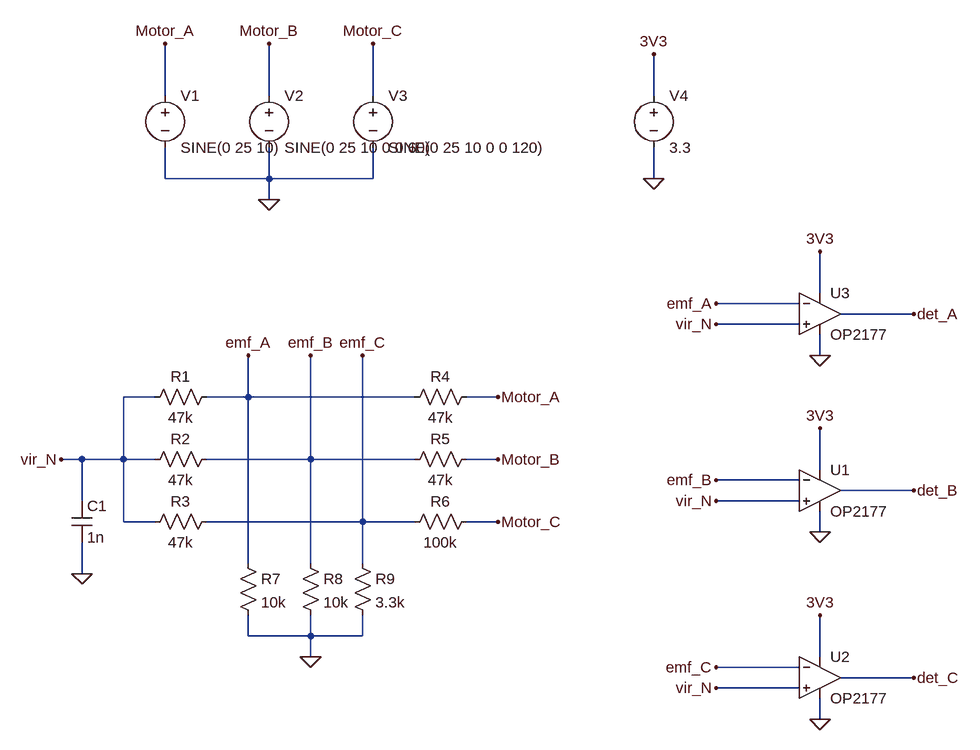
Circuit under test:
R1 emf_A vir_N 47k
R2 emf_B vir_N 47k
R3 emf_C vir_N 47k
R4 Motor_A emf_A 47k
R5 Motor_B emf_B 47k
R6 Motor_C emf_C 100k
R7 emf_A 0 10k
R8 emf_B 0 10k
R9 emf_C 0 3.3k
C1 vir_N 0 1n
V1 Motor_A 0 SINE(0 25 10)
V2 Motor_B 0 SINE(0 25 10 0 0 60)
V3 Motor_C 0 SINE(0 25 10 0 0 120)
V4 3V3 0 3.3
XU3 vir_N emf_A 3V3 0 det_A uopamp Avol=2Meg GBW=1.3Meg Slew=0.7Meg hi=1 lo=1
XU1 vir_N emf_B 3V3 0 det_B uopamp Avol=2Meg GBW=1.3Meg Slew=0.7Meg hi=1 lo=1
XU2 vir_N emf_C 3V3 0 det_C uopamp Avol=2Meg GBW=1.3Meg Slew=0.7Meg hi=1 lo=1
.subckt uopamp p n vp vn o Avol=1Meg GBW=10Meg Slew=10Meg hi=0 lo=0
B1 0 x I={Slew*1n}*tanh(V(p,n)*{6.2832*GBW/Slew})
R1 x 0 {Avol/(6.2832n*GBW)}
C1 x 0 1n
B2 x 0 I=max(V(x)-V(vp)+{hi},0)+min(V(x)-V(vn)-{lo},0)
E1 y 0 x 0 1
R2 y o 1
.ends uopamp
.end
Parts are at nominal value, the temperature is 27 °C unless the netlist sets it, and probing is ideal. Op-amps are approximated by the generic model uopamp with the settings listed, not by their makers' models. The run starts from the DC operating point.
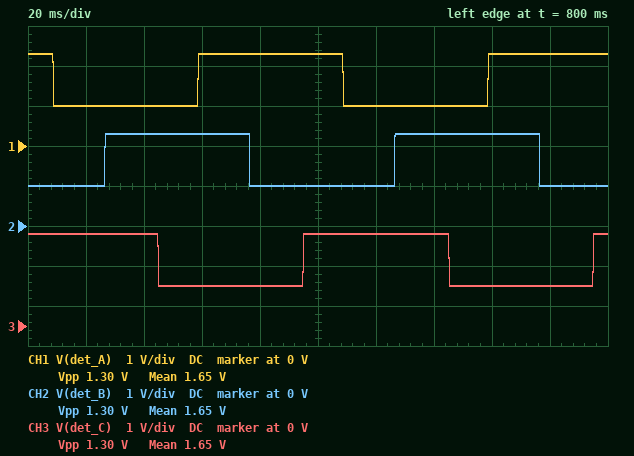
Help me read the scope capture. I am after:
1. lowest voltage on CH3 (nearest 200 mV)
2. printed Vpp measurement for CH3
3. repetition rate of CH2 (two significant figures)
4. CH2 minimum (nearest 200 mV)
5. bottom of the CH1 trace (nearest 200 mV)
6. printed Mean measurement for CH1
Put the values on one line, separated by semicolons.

1.0 V; 1.30 V; 10 Hz; 1.0 V; 1.0 V; 1.65 V
